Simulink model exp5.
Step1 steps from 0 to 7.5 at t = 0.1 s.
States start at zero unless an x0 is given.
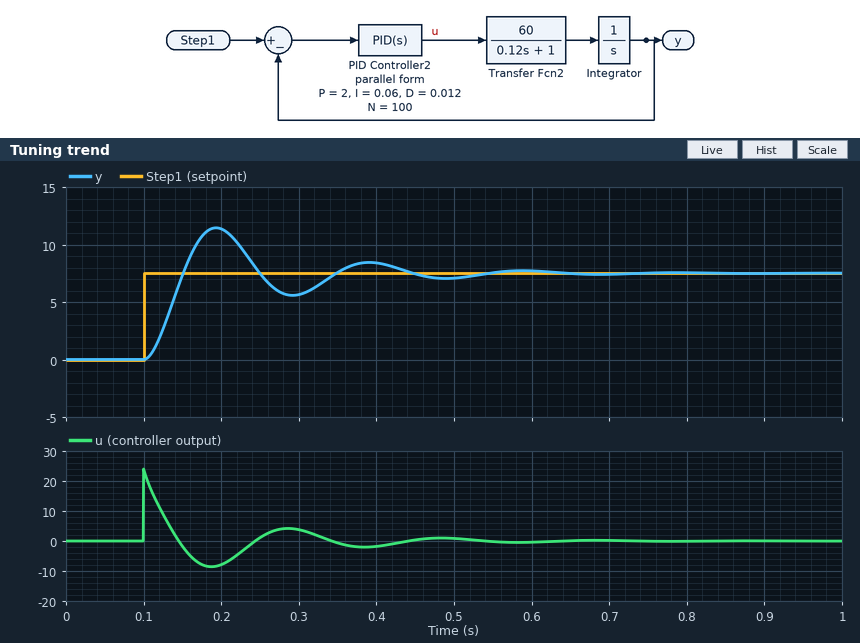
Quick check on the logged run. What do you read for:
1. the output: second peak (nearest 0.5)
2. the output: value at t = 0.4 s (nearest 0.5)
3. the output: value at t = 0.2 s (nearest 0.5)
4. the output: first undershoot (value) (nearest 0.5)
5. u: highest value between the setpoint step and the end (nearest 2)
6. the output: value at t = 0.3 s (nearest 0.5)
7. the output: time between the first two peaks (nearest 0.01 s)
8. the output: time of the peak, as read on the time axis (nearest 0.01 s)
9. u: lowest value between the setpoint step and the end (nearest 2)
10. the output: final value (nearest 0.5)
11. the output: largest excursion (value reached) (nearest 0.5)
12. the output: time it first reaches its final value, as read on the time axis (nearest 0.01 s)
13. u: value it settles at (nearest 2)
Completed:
8.5
8.5
11.5
5.5
24
5.5
0.20 s
0.19 s
-8
7.5
11.5
0.15 s
0
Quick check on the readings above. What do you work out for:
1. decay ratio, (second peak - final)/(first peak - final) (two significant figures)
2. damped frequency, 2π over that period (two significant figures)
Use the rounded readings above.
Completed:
0.25
31 rad/s
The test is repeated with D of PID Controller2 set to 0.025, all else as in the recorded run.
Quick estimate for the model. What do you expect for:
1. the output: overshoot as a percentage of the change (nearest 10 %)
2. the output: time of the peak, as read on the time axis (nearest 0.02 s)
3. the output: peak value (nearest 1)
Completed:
40 %
0.18 s
11
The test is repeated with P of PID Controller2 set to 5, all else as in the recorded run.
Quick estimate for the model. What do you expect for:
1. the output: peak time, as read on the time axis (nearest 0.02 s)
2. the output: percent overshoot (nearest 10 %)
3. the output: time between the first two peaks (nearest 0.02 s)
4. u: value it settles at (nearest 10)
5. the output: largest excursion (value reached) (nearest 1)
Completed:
0.16 s
70 %
0.12 s
0
13
